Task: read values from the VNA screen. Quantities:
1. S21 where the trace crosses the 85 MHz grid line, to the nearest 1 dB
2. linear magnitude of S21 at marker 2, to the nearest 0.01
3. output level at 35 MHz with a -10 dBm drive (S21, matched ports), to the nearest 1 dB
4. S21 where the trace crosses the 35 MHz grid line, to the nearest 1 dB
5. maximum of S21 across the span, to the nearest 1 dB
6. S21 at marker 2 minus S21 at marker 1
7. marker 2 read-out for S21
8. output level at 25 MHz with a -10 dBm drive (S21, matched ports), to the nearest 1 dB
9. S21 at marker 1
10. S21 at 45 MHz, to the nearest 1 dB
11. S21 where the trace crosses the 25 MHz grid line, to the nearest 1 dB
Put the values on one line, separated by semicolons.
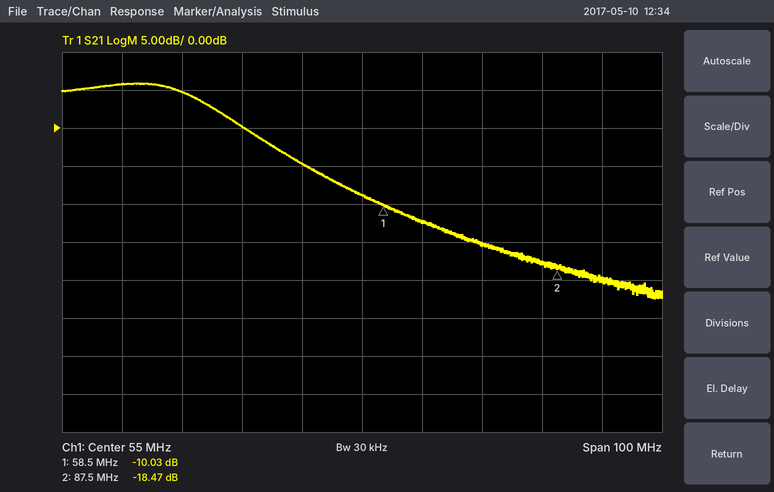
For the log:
-18 dB; 0.12; -10 dBm; 0 dB; 6 dB; -8.44 dB; -18.47 dB; -5 dBm; -10.03 dB; -5 dB; 5 dB
